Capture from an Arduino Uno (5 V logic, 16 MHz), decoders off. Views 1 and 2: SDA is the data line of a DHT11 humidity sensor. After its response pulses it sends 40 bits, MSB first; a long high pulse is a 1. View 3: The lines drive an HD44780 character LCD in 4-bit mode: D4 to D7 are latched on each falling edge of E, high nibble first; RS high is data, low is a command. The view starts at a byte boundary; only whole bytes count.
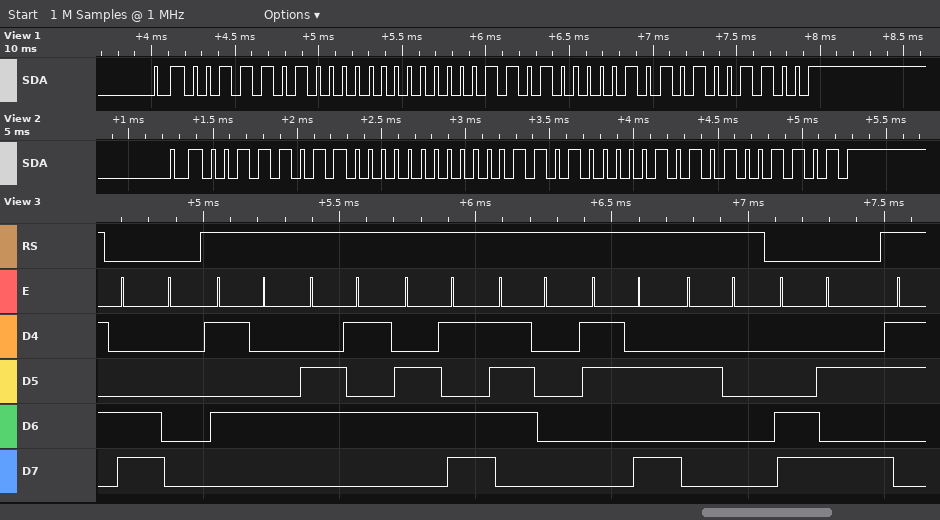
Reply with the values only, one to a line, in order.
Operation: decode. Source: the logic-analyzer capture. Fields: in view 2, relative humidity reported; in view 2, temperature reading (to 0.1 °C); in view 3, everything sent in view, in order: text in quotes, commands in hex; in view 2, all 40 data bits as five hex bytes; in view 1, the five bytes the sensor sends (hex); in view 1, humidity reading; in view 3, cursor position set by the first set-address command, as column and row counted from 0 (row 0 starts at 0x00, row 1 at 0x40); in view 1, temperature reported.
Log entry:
59 %
13.5 °C
0xC0 "Temp: " 0xCA
3B 00 0D 05 4D
3A 00 0D 05 4C
58 %
column 0, row 1
13.5 °C
